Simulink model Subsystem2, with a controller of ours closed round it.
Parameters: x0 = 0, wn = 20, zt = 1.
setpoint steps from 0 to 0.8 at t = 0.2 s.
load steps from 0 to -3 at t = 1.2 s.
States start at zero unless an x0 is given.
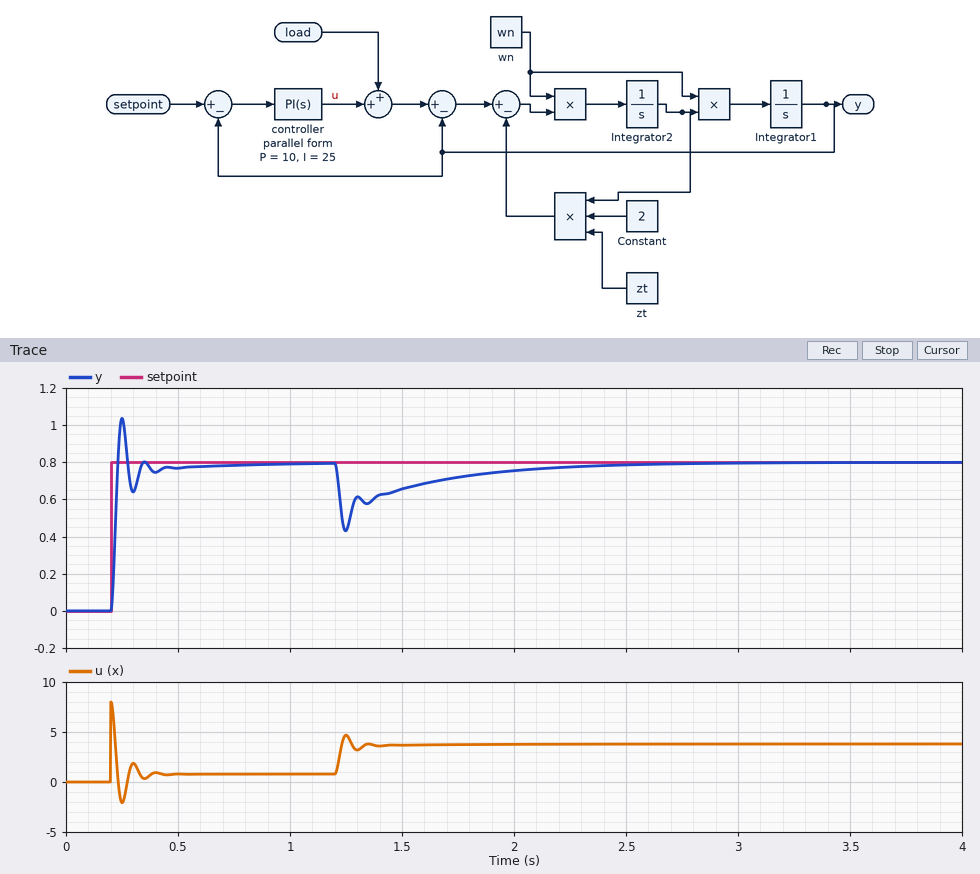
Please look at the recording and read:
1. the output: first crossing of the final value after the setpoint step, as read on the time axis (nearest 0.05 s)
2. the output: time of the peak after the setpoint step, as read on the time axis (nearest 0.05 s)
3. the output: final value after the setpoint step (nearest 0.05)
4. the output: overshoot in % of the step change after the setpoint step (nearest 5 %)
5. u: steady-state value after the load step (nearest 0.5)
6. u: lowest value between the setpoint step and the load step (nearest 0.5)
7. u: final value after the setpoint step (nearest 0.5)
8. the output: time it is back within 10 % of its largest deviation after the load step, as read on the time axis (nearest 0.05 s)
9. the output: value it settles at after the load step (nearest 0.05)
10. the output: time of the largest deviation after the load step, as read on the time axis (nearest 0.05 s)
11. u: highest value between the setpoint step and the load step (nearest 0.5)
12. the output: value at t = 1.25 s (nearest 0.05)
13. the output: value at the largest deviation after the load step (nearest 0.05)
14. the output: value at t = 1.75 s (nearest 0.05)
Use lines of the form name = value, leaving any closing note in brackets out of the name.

the output: first crossing of the final value after the setpoint step, as read on the time axis = 0.25 s
the output: time of the peak after the setpoint step, as read on the time axis = 0.25 s
the output: final value after the setpoint step = 0.80
the output: overshoot in % of the step change after the setpoint step = 30 %
u: steady-state value after the load step = 4.0
u: lowest value between the setpoint step and the load step = -2.0
u: final value after the setpoint step = 1.0
the output: time it is back within 10 % of its largest deviation after the load step, as read on the time axis = 2.10 s
the output: value it settles at after the load step = 0.80
the output: time of the largest deviation after the load step, as read on the time axis = 1.25 s
u: highest value between the setpoint step and the load step = 8.0
the output: value at t = 1.25 s = 0.45
the output: value at the largest deviation after the load step = 0.45
the output: value at t = 1.75 s = 0.70
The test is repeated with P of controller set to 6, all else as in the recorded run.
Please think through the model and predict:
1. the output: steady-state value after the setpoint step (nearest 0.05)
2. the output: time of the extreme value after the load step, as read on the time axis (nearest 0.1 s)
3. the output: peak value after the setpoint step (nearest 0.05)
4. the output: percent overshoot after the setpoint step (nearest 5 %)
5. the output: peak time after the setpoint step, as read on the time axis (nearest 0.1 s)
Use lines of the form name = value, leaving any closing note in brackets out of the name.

the output: steady-state value after the setpoint step = 0.80
the output: time of the extreme value after the load step, as read on the time axis = 1.3 s
the output: peak value after the setpoint step = 0.95
the output: percent overshoot after the setpoint step = 20 %
the output: peak time after the setpoint step, as read on the time axis = 0.3 s
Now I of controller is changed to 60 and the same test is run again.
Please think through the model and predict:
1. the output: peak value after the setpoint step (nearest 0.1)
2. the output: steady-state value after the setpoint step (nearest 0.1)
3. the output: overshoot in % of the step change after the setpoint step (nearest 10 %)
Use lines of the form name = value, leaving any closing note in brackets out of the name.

the output: peak value after the setpoint step = 1.1
the output: steady-state value after the setpoint step = 0.8
the output: overshoot in % of the step change after the setpoint step = 40 %
